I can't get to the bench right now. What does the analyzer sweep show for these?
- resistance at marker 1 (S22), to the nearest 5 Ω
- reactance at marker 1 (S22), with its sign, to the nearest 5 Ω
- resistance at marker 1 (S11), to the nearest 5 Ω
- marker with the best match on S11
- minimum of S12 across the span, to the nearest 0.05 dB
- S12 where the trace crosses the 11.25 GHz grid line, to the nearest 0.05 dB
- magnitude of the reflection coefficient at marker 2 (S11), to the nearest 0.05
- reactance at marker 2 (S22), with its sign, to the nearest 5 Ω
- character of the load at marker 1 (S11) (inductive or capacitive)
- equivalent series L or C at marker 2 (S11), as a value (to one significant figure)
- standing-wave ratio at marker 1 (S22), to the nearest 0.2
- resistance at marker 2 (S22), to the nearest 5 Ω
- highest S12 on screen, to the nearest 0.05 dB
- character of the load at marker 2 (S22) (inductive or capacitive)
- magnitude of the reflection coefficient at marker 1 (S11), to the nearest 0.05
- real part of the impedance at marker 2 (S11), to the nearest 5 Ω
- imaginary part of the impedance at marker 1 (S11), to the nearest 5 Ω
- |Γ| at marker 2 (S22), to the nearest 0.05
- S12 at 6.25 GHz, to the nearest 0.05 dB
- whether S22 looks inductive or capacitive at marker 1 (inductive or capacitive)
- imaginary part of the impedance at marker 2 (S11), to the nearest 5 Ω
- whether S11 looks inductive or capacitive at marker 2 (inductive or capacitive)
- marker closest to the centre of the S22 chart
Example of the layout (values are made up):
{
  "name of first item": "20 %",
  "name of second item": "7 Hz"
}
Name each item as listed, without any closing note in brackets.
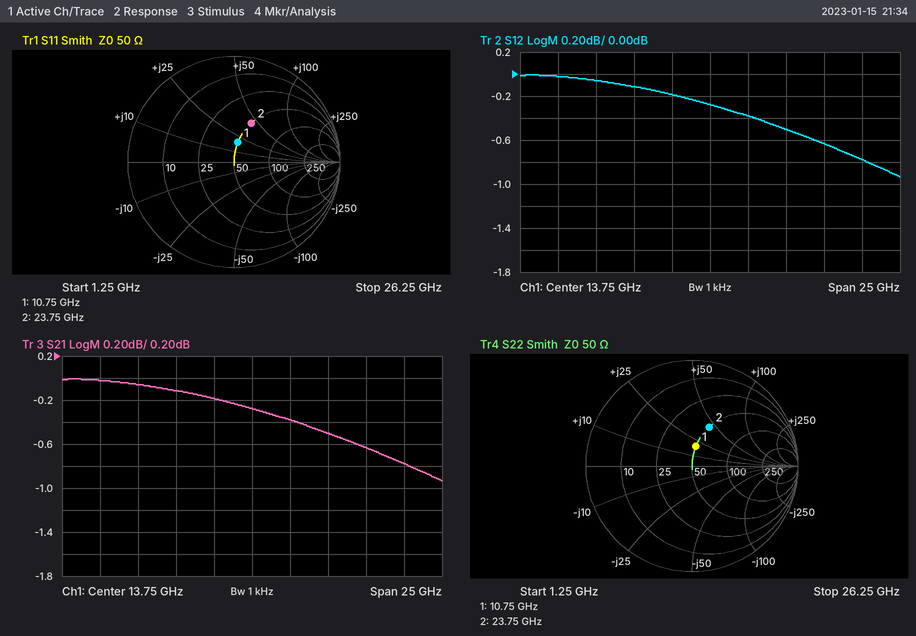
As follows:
{
  "resistance at marker 1 (S22), to the nearest 5 Ω": "50 Ω",
  "reactance at marker 1 (S22), with its sign, to the nearest 5 Ω": "+20 Ω",
  "resistance at marker 1 (S11), to the nearest 5 Ω": "50 Ω",
  "marker with the best match on S11": "marker 1",
  "minimum of S12 across the span, to the nearest 0.05 dB": "-0.95 dB",
  "S12 where the trace crosses the 11.25 GHz grid line, to the nearest 0.05 dB": "-0.20 dB",
  "magnitude of the reflection coefficient at marker 2 (S11), to the nearest 0.05": "0.40",
  "reactance at marker 2 (S22), with its sign, to the nearest 5 Ω": "+45 Ω",
  "character of the load at marker 1 (S11)": "inductive",
  "equivalent series L or C at marker 2 (S11), as a value": "300 pH",
  "standing-wave ratio at marker 1 (S22), to the nearest 0.2": "1.4",
  "resistance at marker 2 (S22), to the nearest 5 Ω": "50 Ω",
  "highest S12 on screen, to the nearest 0.05 dB": "0.00 dB",
  "character of the load at marker 2 (S22)": "inductive",
  "magnitude of the reflection coefficient at marker 1 (S11), to the nearest 0.05": "0.20",
  "real part of the impedance at marker 2 (S11), to the nearest 5 Ω": "50 Ω",
  "imaginary part of the impedance at marker 1 (S11), to the nearest 5 Ω": "+20 Ω",
  "|Γ| at marker 2 (S22), to the nearest 0.05": "0.40",
  "S12 at 6.25 GHz, to the nearest 0.05 dB": "-0.05 dB",
  "whether S22 looks inductive or capacitive at marker 1": "inductive",
  "imaginary part of the impedance at marker 2 (S11), to the nearest 5 Ω": "+45 Ω",
  "whether S11 looks inductive or capacitive at marker 2": "inductive",
  "marker closest to the centre of the S22 chart": "marker 1"
}
